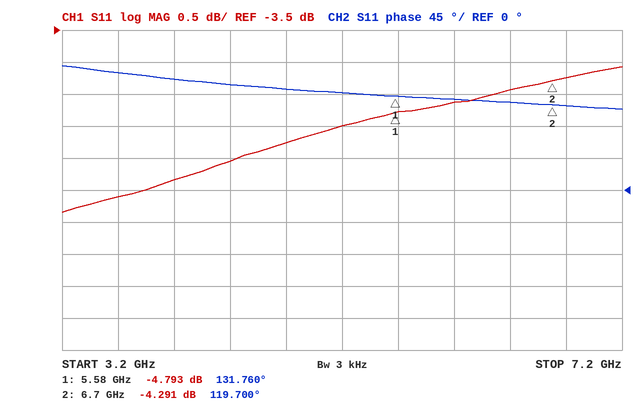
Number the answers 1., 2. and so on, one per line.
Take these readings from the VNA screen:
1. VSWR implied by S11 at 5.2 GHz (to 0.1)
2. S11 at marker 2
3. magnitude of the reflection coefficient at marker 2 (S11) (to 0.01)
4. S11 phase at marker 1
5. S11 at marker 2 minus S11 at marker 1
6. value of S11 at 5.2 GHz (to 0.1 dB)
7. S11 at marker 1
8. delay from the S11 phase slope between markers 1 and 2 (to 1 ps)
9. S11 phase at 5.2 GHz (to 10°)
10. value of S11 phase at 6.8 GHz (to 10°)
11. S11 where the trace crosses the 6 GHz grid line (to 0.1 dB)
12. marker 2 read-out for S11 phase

1. 3.6
2. -4.291 dB
3. 0.61
4. 131.760°
5. 0.502 dB
6. -5.0 dB
7. -4.793 dB
8. 30 ps
9. 140°
10. 120°
11. -4.6 dB
12. 119.700°
